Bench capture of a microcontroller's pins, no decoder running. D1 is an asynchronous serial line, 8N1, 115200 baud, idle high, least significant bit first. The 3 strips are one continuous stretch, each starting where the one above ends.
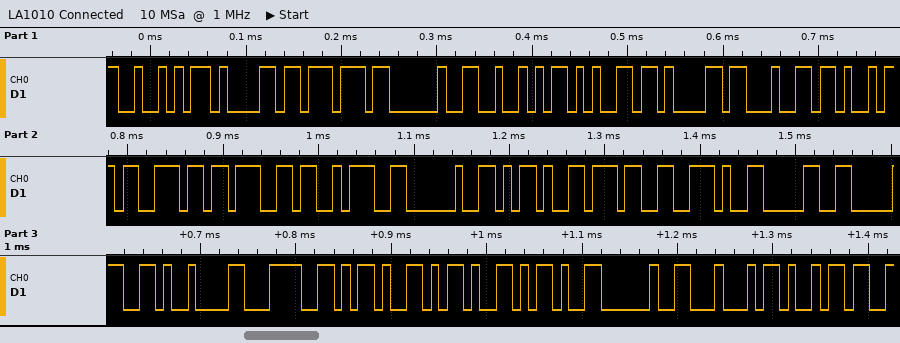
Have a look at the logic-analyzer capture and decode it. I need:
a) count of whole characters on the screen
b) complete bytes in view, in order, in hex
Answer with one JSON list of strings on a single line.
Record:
["26", "52 61 77 20 52 65 61 64 69 6E 67 3A 20 2D 37 2E 30 30 09 3C 2D 2D 2D 20 44 69"]
